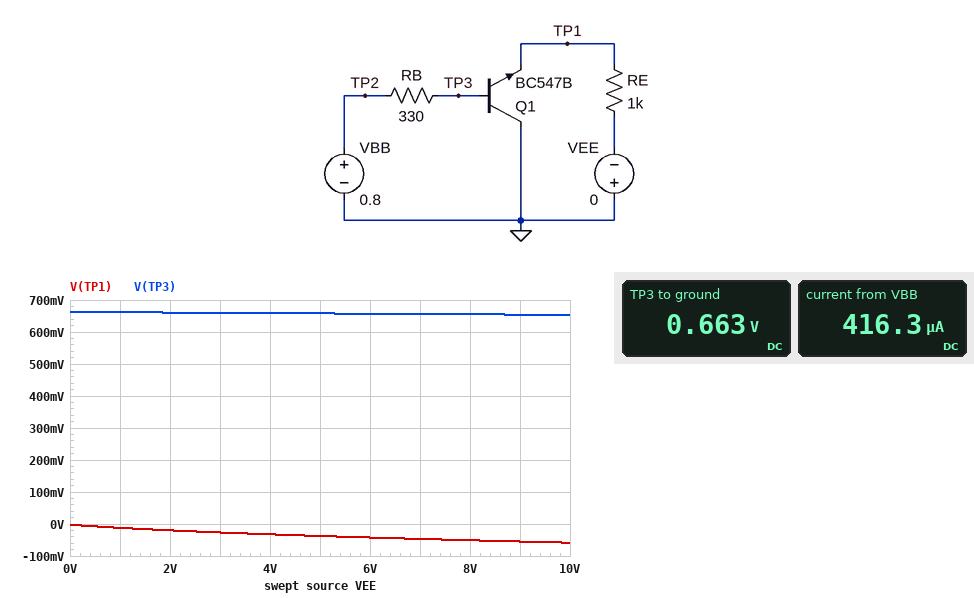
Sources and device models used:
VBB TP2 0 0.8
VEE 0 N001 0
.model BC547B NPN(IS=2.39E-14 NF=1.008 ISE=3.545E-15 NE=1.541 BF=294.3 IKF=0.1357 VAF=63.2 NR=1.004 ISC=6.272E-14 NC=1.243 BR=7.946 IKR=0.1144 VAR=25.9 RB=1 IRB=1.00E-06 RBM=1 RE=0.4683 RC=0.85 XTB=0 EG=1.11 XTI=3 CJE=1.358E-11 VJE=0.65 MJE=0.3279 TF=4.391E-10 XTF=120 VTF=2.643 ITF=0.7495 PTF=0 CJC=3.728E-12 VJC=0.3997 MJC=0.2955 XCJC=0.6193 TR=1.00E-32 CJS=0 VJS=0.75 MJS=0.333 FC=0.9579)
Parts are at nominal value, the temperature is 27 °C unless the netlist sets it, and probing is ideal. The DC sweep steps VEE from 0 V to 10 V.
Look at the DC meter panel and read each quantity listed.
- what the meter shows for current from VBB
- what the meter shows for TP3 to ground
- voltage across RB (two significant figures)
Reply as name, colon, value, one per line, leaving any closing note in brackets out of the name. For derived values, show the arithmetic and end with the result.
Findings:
what the meter shows for current from VBB: 416.3 µA
what the meter shows for TP3 to ground: 0.663 V
voltage across RB: 800 mV - 663 mV = 140 mV
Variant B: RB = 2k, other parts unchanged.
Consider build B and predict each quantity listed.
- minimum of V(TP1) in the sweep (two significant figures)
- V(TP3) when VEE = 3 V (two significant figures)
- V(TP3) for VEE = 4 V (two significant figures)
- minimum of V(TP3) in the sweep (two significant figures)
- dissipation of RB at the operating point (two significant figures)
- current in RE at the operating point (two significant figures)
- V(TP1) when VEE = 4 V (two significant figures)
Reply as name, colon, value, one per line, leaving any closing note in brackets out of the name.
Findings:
minimum of V(TP1) in the sweep: -100 mV
V(TP3) when VEE = 3 V: 620 mV
V(TP3) for VEE = 4 V: 610 mV
minimum of V(TP3) in the sweep: 600 mV
dissipation of RB at the operating point: 16 µW
current in RE at the operating point: 2.2 µA
V(TP1) when VEE = 4 V: -66 mV
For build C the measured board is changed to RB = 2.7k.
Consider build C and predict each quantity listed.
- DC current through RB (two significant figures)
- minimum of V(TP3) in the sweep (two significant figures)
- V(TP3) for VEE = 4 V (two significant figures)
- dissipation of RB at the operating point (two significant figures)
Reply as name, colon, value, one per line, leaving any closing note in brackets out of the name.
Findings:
DC current through RB: 69 µA
minimum of V(TP3) in the sweep: 590 mV
V(TP3) for VEE = 4 V: 610 mV
dissipation of RB at the operating point: 13 µW
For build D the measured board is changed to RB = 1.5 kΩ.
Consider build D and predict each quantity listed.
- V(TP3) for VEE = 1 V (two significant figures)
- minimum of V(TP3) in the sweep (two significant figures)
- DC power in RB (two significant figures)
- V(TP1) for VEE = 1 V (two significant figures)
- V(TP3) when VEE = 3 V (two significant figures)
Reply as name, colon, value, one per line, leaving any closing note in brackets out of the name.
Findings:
V(TP3) for VEE = 1 V: 630 mV
minimum of V(TP3) in the sweep: 610 mV
DC power in RB: 20 µW
V(TP1) for VEE = 1 V: -27 mV
V(TP3) when VEE = 3 V: 620 mV
